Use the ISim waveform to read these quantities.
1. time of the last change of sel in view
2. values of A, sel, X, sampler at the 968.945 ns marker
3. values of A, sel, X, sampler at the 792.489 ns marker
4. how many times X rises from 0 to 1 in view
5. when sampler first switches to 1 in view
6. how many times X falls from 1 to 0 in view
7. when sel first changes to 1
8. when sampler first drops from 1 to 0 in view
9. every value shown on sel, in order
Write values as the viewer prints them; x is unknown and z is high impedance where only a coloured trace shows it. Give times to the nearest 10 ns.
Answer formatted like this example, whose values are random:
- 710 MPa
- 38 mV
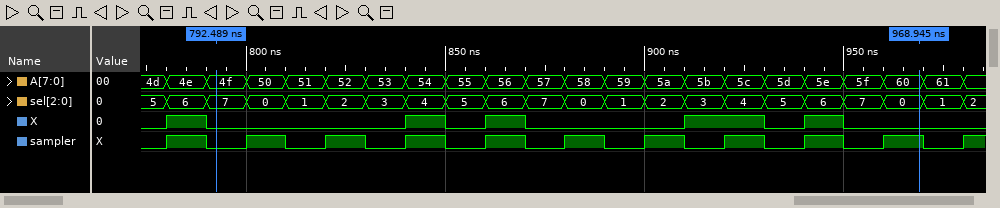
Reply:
- 980 ns
- A=60, sel=0, X=0, sampler=1
- A=4f, sel=7, X=0, sampler=0
- 5
- 780 ns
- 5
- 810 ns
- 790 ns
- 5, 6, 7, 0, 1, 2, 3, 4, 5, 6, 7, 0, 1, 2, 3, 4, 5, 6, 7, 0, 1, 2
